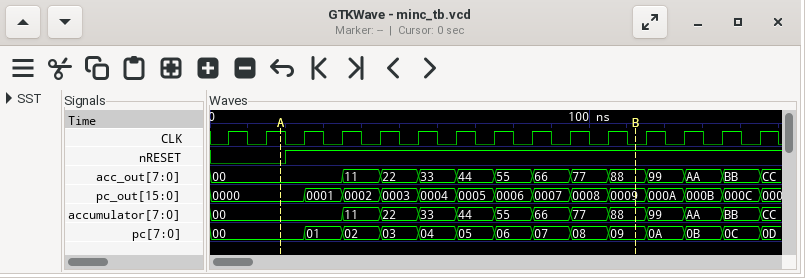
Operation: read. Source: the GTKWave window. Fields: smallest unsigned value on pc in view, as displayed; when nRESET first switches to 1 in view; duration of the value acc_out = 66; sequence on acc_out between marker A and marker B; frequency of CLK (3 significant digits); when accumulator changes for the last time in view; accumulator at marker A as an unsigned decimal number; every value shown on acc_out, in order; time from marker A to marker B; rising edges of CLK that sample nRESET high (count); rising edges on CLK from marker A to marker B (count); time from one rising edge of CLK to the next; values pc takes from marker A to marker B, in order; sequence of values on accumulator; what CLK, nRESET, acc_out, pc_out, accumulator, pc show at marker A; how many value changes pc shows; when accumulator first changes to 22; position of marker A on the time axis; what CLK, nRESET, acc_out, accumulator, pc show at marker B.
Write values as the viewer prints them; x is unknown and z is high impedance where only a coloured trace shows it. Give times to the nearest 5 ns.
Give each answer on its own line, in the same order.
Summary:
00
20 ns
10 ns
00, 11, 22, 33, 44, 55, 66, 77, 88
100 MHz
145 ns
0
00, 11, 22, 33, 44, 55, 66, 77, 88, 99, AA, BB, CC
95 ns
13
9
10 ns
00, 01, 02, 03, 04, 05, 06, 07, 08, 09
00, 11, 22, 33, 44, 55, 66, 77, 88, 99, AA, BB, CC
CLK=1, nRESET=0, acc_out=00, pc_out=0000, accumulator=00, pc=00
13
45 ns
20 ns
CLK=0, nRESET=1, acc_out=88, accumulator=88, pc=09
